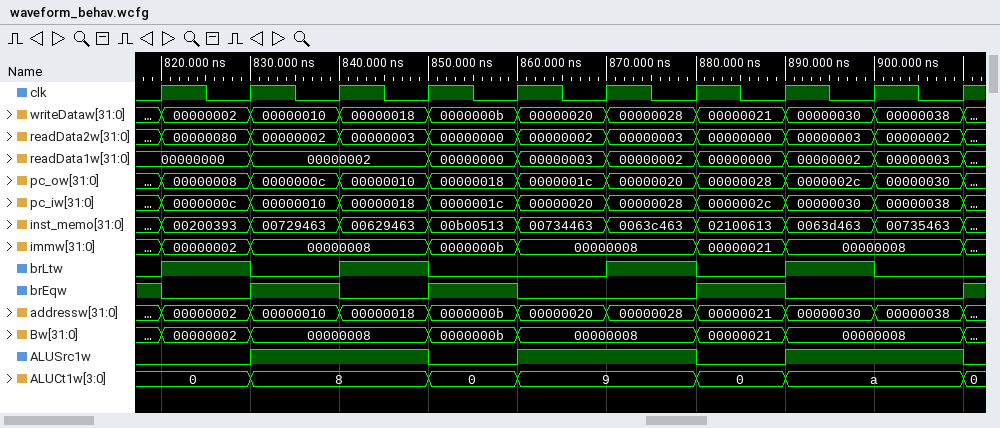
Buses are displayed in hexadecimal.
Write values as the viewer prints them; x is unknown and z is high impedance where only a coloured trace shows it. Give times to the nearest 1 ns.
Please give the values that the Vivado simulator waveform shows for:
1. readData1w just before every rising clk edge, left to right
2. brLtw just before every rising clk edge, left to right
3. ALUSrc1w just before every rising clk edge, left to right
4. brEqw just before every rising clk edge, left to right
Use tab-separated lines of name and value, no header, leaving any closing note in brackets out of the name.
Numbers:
readData1w just before every rising clk edge, left to right	00000000, 00000000, 00000002, 00000002, 00000000, 00000003, 00000002, 00000000, 00000002, 00000003
brLtw just before every rising clk edge, left to right	0 1 0 1 0 0 1 0 1 0
ALUSrc1w just before every rising clk edge, left to right	0 0 1 1 0 1 1 0 1 1
brEqw just before every rising clk edge, left to right	1 0 1 0 1 0 0 1 0 0
